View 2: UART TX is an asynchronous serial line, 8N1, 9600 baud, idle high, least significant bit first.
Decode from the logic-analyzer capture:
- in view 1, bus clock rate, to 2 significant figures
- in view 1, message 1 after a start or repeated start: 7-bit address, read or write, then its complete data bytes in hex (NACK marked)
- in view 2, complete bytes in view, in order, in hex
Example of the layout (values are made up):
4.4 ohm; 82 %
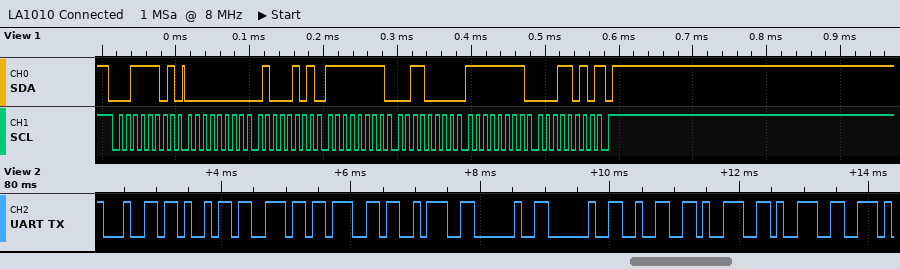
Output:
100 kHz; 0x1E read: 00 45 FF 30 FF 1A NACK; 64 69 6E 67 3A 20 20 32 39 39
